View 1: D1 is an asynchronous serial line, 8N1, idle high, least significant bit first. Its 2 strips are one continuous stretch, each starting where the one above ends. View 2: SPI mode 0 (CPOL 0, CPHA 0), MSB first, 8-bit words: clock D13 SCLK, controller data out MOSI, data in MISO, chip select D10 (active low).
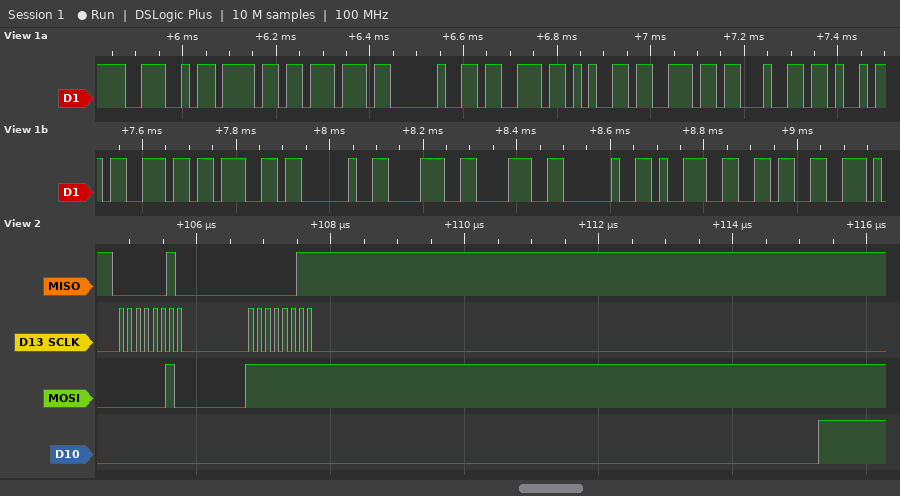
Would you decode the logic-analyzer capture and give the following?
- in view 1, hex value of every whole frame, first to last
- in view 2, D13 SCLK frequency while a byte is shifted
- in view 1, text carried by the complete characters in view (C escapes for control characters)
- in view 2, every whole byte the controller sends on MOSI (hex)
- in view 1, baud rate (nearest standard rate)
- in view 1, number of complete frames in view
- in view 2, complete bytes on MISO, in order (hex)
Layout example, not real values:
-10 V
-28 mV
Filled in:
4E 6F 77 20 73 65 6E 64 69 6E 67 20 38 38 20 39 36
8 MHz
"Now sending 88 96"
02 FF
57600 baud
17
02 03
